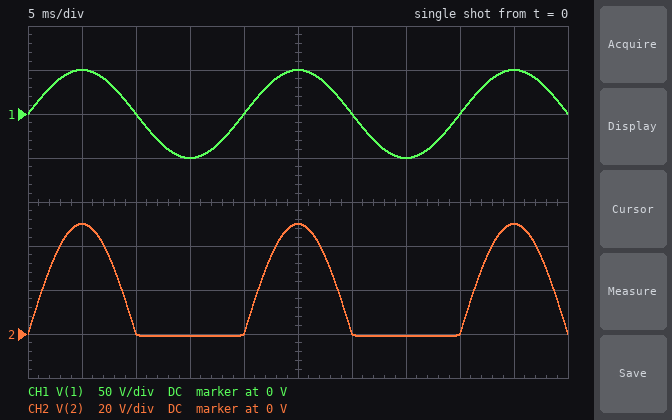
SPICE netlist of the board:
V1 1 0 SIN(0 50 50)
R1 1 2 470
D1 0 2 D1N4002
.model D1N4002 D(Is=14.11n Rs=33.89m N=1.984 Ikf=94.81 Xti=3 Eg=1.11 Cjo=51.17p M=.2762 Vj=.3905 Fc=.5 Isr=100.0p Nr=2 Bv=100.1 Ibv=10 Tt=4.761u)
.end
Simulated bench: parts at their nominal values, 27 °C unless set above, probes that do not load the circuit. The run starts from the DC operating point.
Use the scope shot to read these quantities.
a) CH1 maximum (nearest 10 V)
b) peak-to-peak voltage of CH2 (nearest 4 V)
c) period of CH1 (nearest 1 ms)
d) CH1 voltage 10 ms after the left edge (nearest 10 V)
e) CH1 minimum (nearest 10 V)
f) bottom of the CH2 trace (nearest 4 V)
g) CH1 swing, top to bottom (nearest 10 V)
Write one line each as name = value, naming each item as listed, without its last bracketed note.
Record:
CH1 maximum = 50 V
peak-to-peak voltage of CH2 = 52 V
period of CH1 = 20 ms
CH1 voltage 10 ms after the left edge = 0 V
CH1 minimum = -50 V
bottom of the CH2 trace = 0 V
CH1 swing, top to bottom = 100 V
